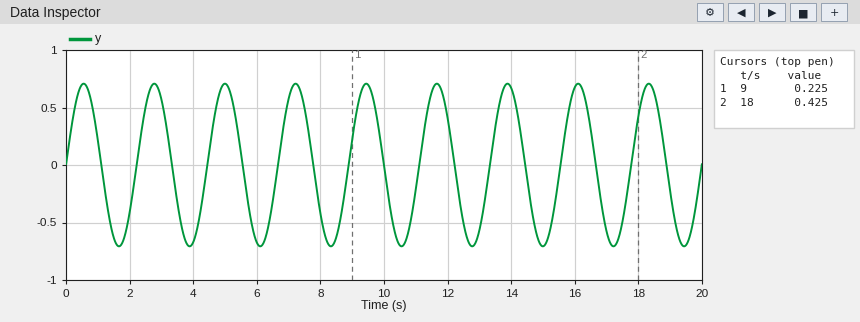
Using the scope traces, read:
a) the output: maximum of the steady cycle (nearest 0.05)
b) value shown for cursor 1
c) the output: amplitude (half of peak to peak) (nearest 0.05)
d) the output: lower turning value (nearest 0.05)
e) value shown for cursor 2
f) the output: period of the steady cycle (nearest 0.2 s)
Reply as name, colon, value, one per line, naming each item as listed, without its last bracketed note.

the output: maximum of the steady cycle: 0.70
value shown for cursor 1: 0.225
the output: amplitude (half of peak to peak): 0.70
the output: lower turning value: -0.70
value shown for cursor 2: 0.425
the output: period of the steady cycle: 2.2 s
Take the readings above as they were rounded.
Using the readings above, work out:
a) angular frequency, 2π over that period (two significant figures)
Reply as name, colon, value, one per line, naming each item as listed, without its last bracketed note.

angular frequency, 2π over that period: 2.9 rad/s
